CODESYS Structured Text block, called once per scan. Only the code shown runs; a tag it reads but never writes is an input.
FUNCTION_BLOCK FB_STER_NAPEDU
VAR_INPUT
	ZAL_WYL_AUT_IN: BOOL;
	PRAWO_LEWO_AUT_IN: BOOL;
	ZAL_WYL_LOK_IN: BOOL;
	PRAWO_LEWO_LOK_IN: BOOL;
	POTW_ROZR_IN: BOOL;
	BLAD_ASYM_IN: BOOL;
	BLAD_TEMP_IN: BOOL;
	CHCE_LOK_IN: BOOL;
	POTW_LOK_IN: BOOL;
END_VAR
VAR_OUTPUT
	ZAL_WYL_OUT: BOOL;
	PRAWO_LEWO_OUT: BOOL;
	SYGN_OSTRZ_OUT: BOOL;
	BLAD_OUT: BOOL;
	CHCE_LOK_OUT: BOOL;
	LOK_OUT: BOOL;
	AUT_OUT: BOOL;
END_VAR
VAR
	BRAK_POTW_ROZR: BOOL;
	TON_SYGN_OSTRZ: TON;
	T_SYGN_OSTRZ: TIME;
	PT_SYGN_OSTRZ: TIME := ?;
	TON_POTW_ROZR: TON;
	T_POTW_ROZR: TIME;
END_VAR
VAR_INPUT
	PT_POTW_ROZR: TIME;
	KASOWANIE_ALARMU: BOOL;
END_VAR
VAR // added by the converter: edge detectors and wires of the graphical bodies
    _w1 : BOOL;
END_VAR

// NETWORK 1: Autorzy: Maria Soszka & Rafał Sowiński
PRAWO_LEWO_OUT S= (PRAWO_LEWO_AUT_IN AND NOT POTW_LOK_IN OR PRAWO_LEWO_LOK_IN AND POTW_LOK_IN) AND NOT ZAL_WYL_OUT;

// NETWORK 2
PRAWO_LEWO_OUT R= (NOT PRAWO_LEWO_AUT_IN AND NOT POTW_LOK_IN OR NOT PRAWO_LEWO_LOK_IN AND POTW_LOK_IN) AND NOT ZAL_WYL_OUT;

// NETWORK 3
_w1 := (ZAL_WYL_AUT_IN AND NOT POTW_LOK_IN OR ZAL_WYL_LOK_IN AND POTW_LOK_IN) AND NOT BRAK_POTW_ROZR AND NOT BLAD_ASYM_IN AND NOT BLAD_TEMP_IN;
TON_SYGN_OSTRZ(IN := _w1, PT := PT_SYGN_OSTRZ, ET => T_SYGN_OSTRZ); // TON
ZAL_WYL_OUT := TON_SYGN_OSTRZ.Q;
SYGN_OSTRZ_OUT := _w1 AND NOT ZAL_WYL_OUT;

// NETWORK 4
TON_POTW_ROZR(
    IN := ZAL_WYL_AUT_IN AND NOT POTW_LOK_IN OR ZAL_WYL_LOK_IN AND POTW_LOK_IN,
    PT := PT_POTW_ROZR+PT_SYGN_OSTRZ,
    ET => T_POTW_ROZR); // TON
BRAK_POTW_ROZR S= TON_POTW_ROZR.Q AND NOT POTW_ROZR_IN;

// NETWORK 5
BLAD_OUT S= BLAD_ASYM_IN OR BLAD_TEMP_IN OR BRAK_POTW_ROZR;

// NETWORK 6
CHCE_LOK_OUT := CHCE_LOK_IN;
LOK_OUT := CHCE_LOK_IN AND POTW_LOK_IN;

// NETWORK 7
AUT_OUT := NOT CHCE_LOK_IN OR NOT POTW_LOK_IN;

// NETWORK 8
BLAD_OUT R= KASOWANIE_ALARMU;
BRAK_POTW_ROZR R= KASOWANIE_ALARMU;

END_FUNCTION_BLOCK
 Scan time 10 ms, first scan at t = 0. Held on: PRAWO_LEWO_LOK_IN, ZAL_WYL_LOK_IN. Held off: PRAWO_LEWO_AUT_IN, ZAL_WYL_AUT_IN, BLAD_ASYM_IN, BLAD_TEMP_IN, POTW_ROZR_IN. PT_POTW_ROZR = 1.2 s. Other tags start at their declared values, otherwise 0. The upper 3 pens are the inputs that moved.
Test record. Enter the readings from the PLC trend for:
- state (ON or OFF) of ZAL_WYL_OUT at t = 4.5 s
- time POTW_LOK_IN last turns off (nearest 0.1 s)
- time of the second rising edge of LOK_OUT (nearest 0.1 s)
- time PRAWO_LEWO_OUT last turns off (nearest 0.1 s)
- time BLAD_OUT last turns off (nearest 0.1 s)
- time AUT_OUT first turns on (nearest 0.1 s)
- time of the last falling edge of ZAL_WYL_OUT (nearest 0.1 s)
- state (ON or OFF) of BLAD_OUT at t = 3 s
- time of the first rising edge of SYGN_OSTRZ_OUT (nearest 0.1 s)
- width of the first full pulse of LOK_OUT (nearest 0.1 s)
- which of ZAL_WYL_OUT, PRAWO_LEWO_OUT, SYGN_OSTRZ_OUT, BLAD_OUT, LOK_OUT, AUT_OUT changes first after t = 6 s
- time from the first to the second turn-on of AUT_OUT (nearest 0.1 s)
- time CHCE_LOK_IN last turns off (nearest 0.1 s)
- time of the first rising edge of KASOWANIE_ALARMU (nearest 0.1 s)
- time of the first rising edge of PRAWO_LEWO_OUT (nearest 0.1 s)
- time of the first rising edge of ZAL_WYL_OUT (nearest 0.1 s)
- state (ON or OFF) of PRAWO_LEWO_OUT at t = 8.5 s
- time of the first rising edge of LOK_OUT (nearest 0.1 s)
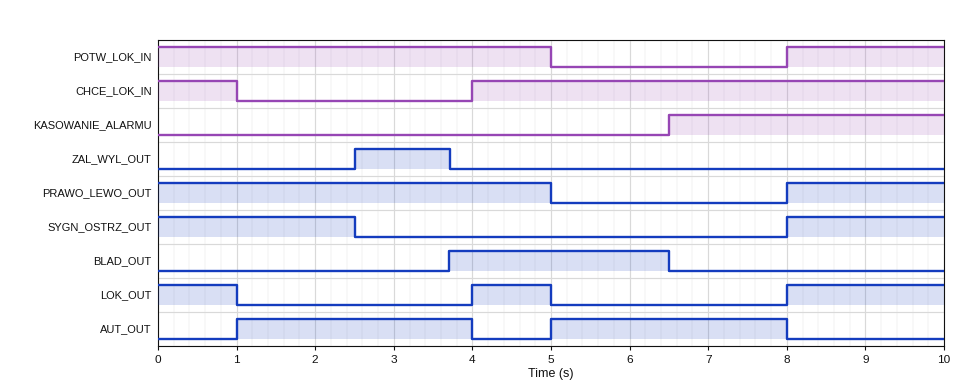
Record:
OFF
5.0 s
8.0 s
5.0 s
6.5 s
1.0 s
3.7 s
OFF
8.0 s
1.0 s
BLAD_OUT
4.0 s
1.0 s
6.5 s
8.0 s
2.5 s
ON
4.0 s
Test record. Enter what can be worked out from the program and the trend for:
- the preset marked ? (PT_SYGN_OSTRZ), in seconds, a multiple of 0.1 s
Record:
2.5 s
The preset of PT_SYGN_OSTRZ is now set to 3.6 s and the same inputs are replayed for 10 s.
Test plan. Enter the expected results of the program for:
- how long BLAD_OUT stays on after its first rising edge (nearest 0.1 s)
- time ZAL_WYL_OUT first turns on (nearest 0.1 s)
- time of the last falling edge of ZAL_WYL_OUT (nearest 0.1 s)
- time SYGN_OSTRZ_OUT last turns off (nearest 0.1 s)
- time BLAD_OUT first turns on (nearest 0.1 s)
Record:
1.7 s
3.6 s
4.8 s
3.6 s
4.8 s
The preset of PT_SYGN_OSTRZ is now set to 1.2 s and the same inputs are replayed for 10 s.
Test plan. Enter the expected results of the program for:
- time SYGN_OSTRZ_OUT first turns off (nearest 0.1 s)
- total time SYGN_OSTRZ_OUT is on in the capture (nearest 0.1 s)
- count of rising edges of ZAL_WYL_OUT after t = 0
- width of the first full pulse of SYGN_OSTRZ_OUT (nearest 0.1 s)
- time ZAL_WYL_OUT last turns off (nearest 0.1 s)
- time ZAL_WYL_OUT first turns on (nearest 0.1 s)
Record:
1.2 s
2.4 s
2
1.2 s
2.4 s
1.2 s
